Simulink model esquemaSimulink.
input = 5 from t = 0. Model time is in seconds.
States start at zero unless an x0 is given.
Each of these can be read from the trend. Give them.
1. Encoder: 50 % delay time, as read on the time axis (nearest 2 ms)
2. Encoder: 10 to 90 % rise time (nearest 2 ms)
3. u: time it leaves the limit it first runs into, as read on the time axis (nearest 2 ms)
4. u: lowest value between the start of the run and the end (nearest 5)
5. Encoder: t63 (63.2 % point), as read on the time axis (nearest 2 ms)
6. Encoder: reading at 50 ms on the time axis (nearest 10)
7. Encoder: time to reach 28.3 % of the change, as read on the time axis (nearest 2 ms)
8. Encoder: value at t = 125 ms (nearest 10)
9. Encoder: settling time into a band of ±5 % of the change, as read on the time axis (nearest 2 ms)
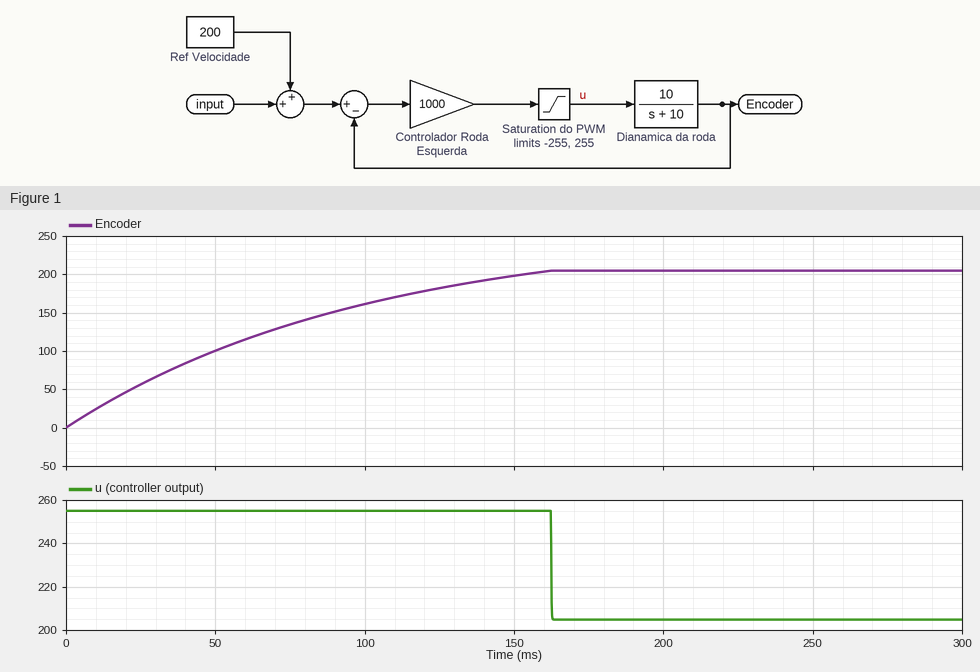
52 ms
120 ms
162 ms
205
70 ms
100
26 ms
180
144 ms
